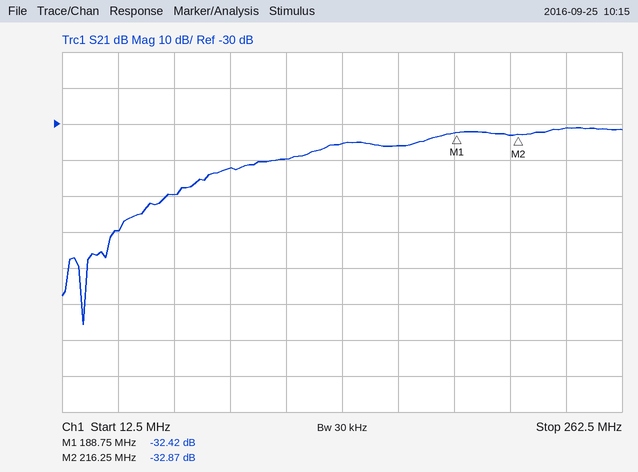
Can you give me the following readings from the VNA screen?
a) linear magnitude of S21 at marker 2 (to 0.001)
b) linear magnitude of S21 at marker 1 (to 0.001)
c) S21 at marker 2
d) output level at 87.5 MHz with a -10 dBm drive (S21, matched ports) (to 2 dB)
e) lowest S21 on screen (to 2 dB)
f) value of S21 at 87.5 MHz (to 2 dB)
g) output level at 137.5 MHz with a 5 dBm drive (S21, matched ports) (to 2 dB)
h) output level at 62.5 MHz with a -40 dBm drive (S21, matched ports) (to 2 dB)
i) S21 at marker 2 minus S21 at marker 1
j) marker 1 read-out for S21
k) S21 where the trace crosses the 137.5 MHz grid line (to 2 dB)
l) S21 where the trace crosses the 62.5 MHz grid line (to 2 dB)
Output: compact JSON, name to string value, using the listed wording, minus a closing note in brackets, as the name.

{"linear magnitude of S21 at marker 2": "0.023", "linear magnitude of S21 at marker 1": "0.024", "S21 at marker 2": "-32.87 dB", "output level at 87.5 MHz with a -10 dBm drive (S21, matched ports)": "-52 dBm", "lowest S21 on screen": "-86 dB", "value of S21 at 87.5 MHz": "-42 dB", "output level at 137.5 MHz with a 5 dBm drive (S21, matched ports)": "-30 dBm", "output level at 62.5 MHz with a -40 dBm drive (S21, matched ports)": "-90 dBm", "S21 at marker 2 minus S21 at marker 1": "-0.45 dB", "marker 1 read-out for S21": "-32.42 dB", "S21 where the trace crosses the 137.5 MHz grid line": "-36 dB", "S21 where the trace crosses the 62.5 MHz grid line": "-50 dB"}
